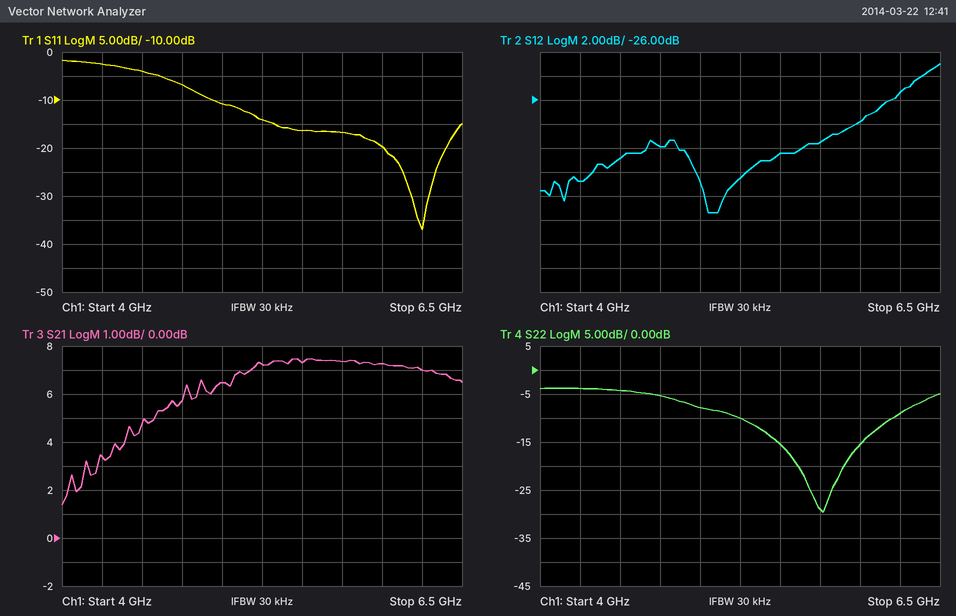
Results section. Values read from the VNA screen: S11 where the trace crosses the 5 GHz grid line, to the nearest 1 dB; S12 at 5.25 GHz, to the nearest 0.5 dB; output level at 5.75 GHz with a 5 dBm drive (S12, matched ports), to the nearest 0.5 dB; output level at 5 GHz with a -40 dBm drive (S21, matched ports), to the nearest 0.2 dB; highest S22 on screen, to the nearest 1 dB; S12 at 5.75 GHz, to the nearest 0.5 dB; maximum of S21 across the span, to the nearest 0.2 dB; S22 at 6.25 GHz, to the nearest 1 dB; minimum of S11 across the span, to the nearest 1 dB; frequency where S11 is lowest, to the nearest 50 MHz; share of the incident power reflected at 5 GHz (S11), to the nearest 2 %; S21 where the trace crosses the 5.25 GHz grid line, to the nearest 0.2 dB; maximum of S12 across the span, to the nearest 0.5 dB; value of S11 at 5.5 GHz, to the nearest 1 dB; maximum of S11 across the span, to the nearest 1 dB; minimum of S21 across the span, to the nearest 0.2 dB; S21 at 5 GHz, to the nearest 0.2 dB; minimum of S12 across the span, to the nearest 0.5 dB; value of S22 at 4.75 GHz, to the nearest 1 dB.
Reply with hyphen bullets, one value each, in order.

- -11 dB
- -32.5 dB
- -24.5 dBm
- -33.6 dBm
- -4 dB
- -29.5 dB
- 7.4 dB
- -9 dB
- -37 dB
- 6.25 GHz
- 8 %
- 7.2 dB
- -23.0 dB
- -16 dB
- -2 dB
- 1.4 dB
- 6.4 dB
- -35.5 dB
- -5 dB
